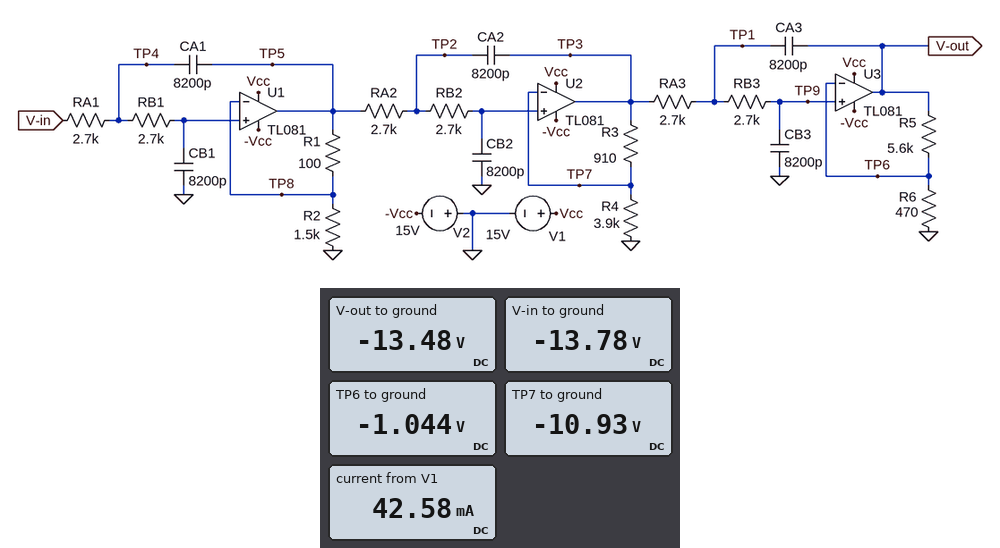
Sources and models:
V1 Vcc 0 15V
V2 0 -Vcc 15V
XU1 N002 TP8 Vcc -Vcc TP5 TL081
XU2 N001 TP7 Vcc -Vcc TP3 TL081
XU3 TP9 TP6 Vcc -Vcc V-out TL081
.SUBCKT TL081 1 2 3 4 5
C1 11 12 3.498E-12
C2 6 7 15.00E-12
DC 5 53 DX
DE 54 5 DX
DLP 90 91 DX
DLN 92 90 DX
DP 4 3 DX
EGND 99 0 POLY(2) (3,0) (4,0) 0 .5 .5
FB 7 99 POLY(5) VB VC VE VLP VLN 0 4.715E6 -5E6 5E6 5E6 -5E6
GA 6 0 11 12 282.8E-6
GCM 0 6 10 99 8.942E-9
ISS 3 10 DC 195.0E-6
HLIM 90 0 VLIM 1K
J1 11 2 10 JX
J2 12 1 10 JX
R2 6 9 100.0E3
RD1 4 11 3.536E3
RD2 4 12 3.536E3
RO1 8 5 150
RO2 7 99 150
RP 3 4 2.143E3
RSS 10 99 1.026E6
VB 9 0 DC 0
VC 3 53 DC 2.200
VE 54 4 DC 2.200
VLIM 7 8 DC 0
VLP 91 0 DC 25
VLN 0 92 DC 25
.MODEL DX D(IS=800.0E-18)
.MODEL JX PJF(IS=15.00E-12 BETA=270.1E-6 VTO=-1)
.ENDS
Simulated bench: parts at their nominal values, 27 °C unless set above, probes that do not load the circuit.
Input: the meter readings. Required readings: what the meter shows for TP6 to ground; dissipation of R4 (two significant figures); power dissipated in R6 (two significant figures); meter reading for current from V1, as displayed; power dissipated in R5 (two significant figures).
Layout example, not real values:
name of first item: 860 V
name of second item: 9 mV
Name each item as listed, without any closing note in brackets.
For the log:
what the meter shows for TP6 to ground: -1.044 V
dissipation of R4: 31 mW
power dissipated in R6: 2.3 mW
meter reading for current from V1, as displayed: 42.58 mA
power dissipated in R5: 28 mW
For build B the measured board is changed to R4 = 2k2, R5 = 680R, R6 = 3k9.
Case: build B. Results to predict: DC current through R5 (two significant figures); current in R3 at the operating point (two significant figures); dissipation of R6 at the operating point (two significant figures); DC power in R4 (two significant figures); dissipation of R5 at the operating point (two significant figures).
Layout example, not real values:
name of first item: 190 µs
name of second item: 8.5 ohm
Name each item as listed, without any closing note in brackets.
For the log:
DC current through R5: 2.9 mA
current in R3 at the operating point: 4.3 mA
dissipation of R6 at the operating point: 34 mW
DC power in R4: 41 mW
dissipation of R5 at the operating point: 5.9 mW
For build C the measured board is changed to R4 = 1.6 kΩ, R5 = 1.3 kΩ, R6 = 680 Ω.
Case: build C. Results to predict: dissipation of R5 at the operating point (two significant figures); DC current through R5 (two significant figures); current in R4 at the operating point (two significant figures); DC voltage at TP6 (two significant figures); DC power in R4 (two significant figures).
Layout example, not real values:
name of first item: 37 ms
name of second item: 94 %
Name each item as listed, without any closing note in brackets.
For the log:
dissipation of R5 at the operating point: 60 mW
DC current through R5: 6.8 mA
current in R4 at the operating point: 5.4 mA
DC voltage at TP6: -4.6 V
DC power in R4: 46 mW
